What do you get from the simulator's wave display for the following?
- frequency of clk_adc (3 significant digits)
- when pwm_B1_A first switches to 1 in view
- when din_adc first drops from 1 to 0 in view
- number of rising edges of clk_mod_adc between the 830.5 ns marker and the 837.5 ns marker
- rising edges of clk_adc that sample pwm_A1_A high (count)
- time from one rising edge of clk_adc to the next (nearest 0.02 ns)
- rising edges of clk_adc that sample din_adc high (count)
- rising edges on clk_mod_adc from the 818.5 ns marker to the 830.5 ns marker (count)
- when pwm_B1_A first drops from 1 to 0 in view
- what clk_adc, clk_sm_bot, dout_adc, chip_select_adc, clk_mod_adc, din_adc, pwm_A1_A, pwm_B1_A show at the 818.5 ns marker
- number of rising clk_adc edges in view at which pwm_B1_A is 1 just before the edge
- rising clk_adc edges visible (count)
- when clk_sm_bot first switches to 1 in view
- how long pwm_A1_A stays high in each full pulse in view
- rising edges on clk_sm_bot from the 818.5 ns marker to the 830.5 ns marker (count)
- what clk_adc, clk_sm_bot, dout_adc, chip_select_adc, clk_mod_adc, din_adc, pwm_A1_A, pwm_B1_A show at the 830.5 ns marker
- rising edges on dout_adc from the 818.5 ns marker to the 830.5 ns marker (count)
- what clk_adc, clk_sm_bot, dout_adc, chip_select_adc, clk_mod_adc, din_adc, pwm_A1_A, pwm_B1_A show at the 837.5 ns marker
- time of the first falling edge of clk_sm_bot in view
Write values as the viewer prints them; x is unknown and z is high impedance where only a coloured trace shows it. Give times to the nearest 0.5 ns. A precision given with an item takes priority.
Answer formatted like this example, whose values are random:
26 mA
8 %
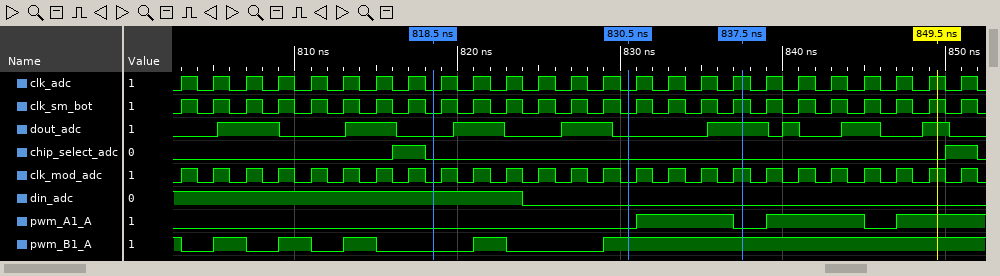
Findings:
500 MHz
805 ns
824 ns
4
8
2 ns
11
6
803 ns
clk_adc=0, clk_sm_bot=0, dout_adc=0, chip_select_adc=0, clk_mod_adc=0, din_adc=1, pwm_A1_A=0, pwm_B1_A=0
16
25
803 ns
6 ns, 6 ns
6
clk_adc=0, clk_sm_bot=0, dout_adc=0, chip_select_adc=0, clk_mod_adc=0, din_adc=0, pwm_A1_A=0, pwm_B1_A=1
2
clk_adc=1, clk_sm_bot=1, dout_adc=1, chip_select_adc=0, clk_mod_adc=1, din_adc=0, pwm_A1_A=0, pwm_B1_A=1
804 ns
